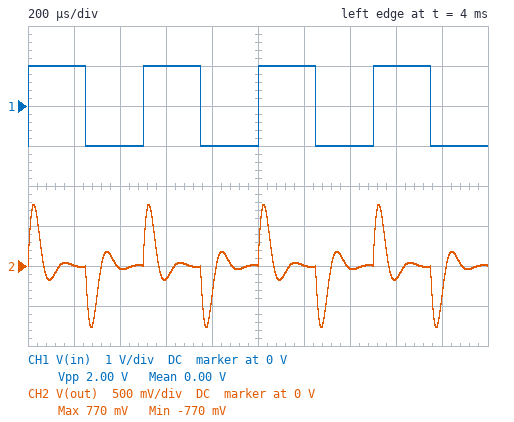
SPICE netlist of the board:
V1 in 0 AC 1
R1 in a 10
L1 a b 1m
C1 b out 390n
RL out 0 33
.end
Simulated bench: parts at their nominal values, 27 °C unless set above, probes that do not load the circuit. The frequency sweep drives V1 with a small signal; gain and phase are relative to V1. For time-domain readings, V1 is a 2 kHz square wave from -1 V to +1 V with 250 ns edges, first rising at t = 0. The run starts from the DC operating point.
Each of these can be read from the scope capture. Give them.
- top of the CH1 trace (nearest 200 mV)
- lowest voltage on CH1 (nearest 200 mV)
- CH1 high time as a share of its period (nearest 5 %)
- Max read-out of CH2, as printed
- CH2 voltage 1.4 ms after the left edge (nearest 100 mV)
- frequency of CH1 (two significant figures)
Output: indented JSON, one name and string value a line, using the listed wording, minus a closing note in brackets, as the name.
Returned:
{
  "top of the CH1 trace": "1.0 V",
  "lowest voltage on CH1": "-1.0 V",
  "CH1 high time as a share of its period": "50 %",
  "Max read-out of CH2, as printed": "770 mV",
  "CH2 voltage 1.4 ms after the left edge": "0 V",
  "frequency of CH1": "2.0 kHz"
}
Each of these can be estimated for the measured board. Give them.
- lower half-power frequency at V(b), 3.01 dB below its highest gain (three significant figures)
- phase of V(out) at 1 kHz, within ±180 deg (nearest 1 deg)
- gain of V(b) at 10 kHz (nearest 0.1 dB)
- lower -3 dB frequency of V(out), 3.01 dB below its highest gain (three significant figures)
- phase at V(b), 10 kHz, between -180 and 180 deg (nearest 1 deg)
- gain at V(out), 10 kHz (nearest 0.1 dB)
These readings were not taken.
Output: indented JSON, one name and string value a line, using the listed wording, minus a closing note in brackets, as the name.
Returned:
{
  "lower half-power frequency at V(b), 3.01 dB below its highest gain": "1.85 kHz",
  "phase of V(out) at 1 kHz, within ±180 deg": "84 deg",
  "gain of V(b) at 10 kHz": "0.7 dB",
  "lower -3 dB frequency of V(out), 3.01 dB below its highest gain": "5.33 kHz",
  "phase at V(b), 10 kHz, between -180 and 180 deg": "-78 deg",
  "gain at V(out), 10 kHz": "-3.3 dB"
}
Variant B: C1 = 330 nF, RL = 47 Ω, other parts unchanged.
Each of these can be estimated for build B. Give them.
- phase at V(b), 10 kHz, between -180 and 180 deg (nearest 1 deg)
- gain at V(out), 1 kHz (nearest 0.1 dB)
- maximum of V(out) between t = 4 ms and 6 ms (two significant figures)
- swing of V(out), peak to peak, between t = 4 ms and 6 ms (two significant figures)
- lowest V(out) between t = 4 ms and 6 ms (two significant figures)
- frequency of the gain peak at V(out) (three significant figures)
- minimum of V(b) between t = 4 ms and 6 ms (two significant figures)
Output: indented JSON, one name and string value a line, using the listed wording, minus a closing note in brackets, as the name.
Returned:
{
  "phase at V(b), 10 kHz, between -180 and 180 deg": "-60 deg",
  "gain at V(out), 1 kHz": "-20.2 dB",
  "maximum of V(out) between t = 4 ms and 6 ms": "920 mV",
  "swing of V(out), peak to peak, between t = 4 ms and 6 ms": "1.8 V",
  "lowest V(out) between t = 4 ms and 6 ms": "-920 mV",
  "frequency of the gain peak at V(out)": "8.76 kHz",
  "minimum of V(b) between t = 4 ms and 6 ms": "-1.5 V"
}
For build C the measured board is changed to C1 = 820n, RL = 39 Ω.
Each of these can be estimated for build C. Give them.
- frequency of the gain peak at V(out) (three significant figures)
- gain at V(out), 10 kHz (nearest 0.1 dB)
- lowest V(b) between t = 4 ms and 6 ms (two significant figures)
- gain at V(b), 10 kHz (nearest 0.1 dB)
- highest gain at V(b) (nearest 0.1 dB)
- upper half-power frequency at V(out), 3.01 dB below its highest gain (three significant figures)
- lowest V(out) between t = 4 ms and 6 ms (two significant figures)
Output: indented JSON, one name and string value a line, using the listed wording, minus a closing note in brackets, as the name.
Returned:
{
  "frequency of the gain peak at V(out)": "5.56 kHz",
  "gain at V(out), 10 kHz": "-4.5 dB",
  "lowest V(b) between t = 4 ms and 6 ms": "-1.3 V",
  "gain at V(b), 10 kHz": "-3.5 dB",
  "highest gain at V(b)": "1.2 dB",
  "upper half-power frequency at V(out), 3.01 dB below its highest gain": "10.7 kHz",
  "lowest V(out) between t = 4 ms and 6 ms": "-1.0 V"
}
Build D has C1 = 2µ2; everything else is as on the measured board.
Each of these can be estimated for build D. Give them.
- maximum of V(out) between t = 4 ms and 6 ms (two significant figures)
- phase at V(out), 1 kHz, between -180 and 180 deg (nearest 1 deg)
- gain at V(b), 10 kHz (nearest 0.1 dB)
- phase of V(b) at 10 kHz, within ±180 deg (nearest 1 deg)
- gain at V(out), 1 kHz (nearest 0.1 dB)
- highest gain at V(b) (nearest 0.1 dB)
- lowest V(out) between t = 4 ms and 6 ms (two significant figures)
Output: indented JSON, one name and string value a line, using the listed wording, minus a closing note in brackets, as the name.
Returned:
{
  "maximum of V(out) between t = 4 ms and 6 ms": "1.1 V",
  "phase at V(out), 1 kHz, between -180 and 180 deg": "57 deg",
  "gain at V(b), 10 kHz": "-6.4 dB",
  "phase of V(b) at 10 kHz, within ±180 deg": "-65 deg",
  "gain at V(out), 1 kHz": "-7.6 dB",
  "highest gain at V(b)": "0.1 dB",
  "lowest V(out) between t = 4 ms and 6 ms": "-1.1 V"
}
